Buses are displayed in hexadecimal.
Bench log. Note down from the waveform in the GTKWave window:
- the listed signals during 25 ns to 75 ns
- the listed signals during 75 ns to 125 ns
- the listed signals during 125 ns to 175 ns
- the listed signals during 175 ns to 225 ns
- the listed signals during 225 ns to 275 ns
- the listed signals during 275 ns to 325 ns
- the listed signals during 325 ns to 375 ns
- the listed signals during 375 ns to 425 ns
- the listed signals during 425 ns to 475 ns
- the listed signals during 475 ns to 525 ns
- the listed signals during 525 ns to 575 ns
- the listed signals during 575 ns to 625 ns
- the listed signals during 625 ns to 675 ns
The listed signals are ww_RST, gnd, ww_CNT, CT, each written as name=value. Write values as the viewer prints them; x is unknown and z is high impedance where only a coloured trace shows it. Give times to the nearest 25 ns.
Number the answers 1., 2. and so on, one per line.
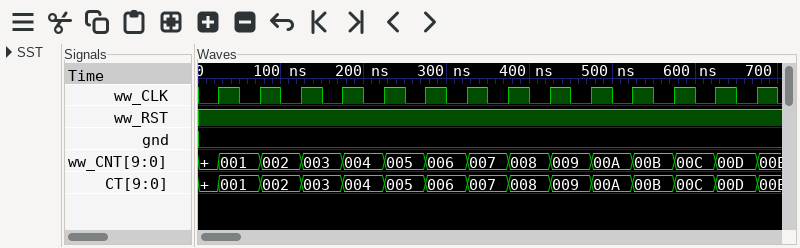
1. ww_RST=1, gnd=0, ww_CNT=001, CT=001
2. ww_RST=1, gnd=0, ww_CNT=002, CT=002
3. ww_RST=1, gnd=0, ww_CNT=003, CT=003
4. ww_RST=1, gnd=0, ww_CNT=004, CT=004
5. ww_RST=1, gnd=0, ww_CNT=005, CT=005
6. ww_RST=1, gnd=0, ww_CNT=006, CT=006
7. ww_RST=1, gnd=0, ww_CNT=007, CT=007
8. ww_RST=1, gnd=0, ww_CNT=008, CT=008
9. ww_RST=1, gnd=0, ww_CNT=009, CT=009
10. ww_RST=1, gnd=0, ww_CNT=00A, CT=00A
11. ww_RST=1, gnd=0, ww_CNT=00B, CT=00B
12. ww_RST=1, gnd=0, ww_CNT=00C, CT=00C
13. ww_RST=1, gnd=0, ww_CNT=00D, CT=00D
